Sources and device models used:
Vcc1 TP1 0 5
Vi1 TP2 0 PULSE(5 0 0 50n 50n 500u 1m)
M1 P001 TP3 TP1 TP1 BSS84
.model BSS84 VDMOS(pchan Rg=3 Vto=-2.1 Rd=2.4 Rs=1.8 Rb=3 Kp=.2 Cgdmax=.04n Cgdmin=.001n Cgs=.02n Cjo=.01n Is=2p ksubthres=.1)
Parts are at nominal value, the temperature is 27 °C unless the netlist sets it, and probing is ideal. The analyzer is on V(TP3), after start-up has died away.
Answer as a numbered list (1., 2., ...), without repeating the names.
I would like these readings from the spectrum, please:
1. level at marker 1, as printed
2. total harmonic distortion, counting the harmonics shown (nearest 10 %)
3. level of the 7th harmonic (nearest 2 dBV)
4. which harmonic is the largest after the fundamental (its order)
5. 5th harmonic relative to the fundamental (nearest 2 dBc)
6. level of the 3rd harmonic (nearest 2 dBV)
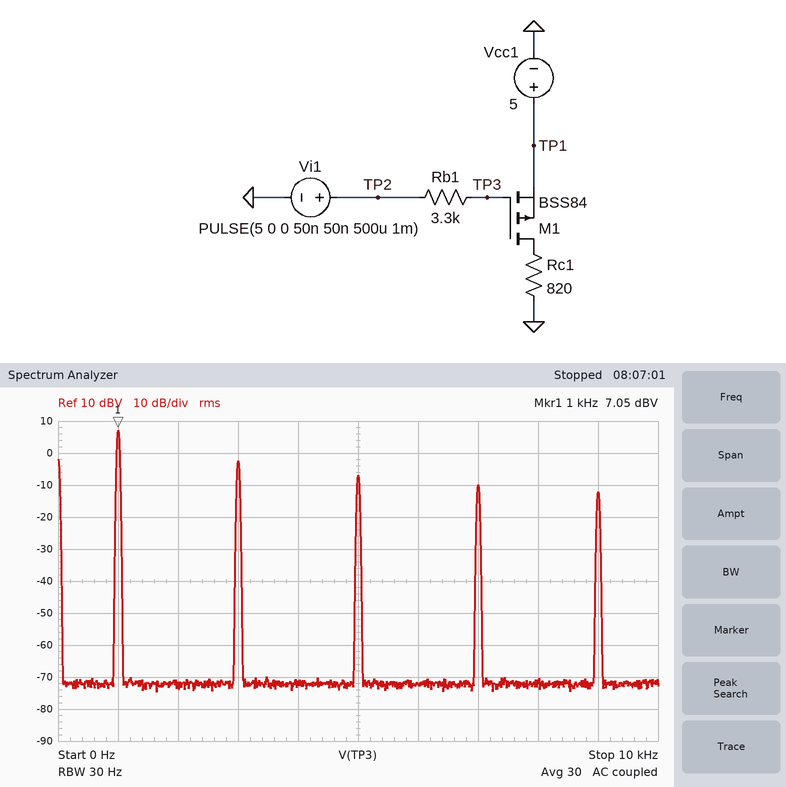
1. 7.05 dBV
2. 40 %
3. -10 dBV
4. 3
5. -14 dBc
6. -2 dBV
